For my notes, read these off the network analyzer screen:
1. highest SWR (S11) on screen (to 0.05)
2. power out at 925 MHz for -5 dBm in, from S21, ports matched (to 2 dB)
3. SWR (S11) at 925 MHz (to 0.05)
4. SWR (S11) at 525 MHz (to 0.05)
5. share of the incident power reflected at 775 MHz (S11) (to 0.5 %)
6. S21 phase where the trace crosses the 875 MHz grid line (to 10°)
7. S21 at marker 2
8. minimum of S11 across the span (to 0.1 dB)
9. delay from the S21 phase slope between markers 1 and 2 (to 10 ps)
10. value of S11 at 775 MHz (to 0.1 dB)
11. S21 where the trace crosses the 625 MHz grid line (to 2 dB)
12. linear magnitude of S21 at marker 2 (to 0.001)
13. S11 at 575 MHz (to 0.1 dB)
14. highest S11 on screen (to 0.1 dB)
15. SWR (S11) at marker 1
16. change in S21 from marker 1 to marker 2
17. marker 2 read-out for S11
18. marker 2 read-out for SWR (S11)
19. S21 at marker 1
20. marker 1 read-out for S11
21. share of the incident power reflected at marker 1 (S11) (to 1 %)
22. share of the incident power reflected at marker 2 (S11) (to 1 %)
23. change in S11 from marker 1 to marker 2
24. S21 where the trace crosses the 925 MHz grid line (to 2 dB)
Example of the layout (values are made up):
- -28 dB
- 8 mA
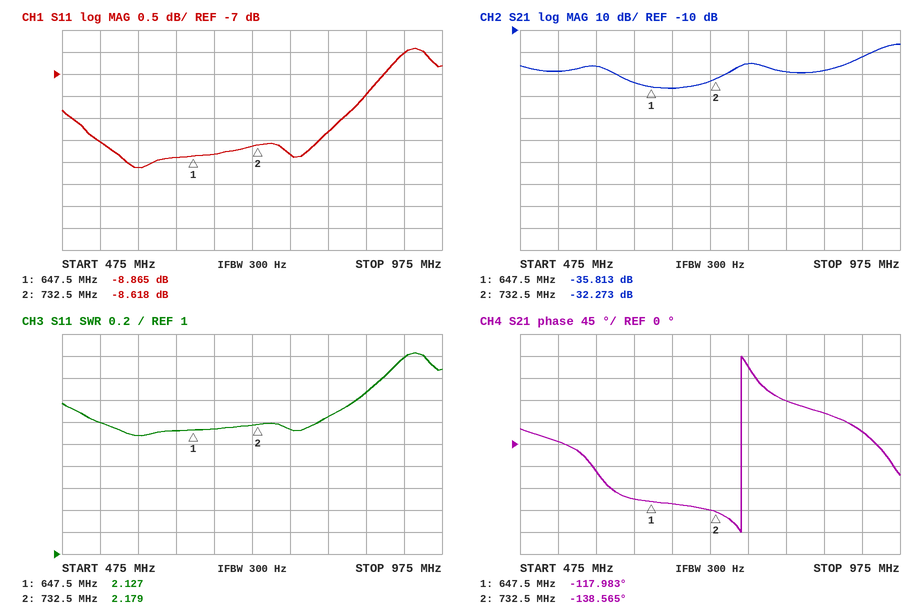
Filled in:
- 2.85
- -28 dBm
- 2.80
- 2.20
- 13.0 %
- 60°
- -32.273 dB
- -9.1 dB
- 670 ps
- -8.8 dB
- -34 dB
- 0.024
- -9.1 dB
- -6.4 dB
- 2.127
- 3.540 dB
- -8.618 dB
- 2.179
- -35.813 dB
- -8.865 dB
- 13 %
- 14 %
- 0.247 dB
- -22 dB
